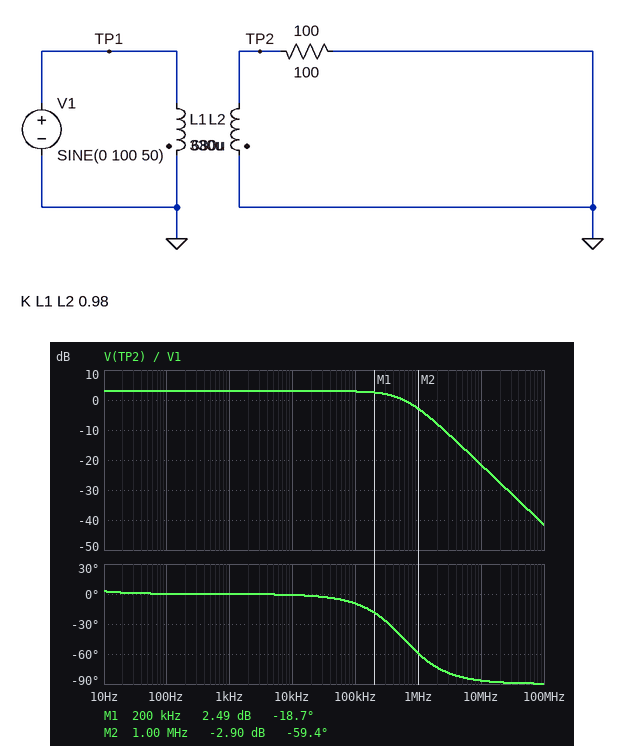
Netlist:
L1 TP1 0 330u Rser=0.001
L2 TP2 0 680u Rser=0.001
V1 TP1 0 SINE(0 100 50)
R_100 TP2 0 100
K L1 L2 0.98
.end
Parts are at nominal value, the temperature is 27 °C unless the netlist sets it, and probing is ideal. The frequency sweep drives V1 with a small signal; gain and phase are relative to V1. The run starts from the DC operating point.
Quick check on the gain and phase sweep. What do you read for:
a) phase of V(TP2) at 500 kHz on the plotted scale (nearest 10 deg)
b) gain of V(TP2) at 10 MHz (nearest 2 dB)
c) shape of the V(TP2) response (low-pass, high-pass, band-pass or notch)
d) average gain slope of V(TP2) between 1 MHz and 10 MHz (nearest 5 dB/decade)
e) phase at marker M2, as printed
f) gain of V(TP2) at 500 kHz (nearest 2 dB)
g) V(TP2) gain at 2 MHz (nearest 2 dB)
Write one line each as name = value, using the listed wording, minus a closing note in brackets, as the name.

phase of V(TP2) at 500 kHz on the plotted scale = -40 deg
gain of V(TP2) at 10 MHz = -22 dB
shape of the V(TP2) response = low-pass
average gain slope of V(TP2) between 1 MHz and 10 MHz = -20 dB/decade
phase at marker M2, as printed = -59.4 deg
gain of V(TP2) at 500 kHz = 0 dB
V(TP2) gain at 2 MHz = -8 dB
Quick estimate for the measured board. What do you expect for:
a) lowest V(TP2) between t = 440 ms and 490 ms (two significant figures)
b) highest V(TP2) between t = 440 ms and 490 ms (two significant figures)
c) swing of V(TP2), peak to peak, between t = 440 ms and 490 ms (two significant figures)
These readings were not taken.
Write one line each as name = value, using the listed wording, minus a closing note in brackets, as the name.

lowest V(TP2) between t = 440 ms and 490 ms = -140 V
highest V(TP2) between t = 440 ms and 490 ms = 140 V
swing of V(TP2), peak to peak, between t = 440 ms and 490 ms = 280 V
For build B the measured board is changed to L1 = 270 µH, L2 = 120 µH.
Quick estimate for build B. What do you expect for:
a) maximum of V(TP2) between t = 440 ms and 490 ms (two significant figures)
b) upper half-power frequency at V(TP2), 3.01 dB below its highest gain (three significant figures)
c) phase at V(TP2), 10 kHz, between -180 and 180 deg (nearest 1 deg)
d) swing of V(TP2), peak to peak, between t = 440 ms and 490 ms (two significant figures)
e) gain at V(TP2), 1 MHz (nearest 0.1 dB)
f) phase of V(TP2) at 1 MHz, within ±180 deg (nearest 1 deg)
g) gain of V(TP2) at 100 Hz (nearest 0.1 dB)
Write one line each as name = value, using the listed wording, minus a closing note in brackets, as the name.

maximum of V(TP2) between t = 440 ms and 490 ms = 65 V
upper half-power frequency at V(TP2), 3.01 dB below its highest gain = 3.35 MHz
phase at V(TP2), 10 kHz, between -180 and 180 deg = 0 deg
swing of V(TP2), peak to peak, between t = 440 ms and 490 ms = 130 V
gain at V(TP2), 1 MHz = -4.1 dB
phase of V(TP2) at 1 MHz, within ±180 deg = -17 deg
gain of V(TP2) at 100 Hz = -3.7 dB
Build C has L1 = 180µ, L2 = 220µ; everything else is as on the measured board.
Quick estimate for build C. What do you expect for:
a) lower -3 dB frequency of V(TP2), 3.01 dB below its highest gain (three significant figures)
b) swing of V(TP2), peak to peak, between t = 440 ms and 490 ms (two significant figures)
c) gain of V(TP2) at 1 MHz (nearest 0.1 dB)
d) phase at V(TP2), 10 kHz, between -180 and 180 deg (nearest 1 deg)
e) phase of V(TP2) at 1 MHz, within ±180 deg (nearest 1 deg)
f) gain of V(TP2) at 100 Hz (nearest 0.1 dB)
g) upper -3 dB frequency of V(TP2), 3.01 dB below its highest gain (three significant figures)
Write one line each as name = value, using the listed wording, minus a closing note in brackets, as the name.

lower -3 dB frequency of V(TP2), 3.01 dB below its highest gain = 884 mHz
swing of V(TP2), peak to peak, between t = 440 ms and 490 ms = 220 V
gain of V(TP2) at 1 MHz = -0.4 dB
phase at V(TP2), 10 kHz, between -180 and 180 deg = 0 deg
phase of V(TP2) at 1 MHz, within ±180 deg = -29 deg
gain of V(TP2) at 100 Hz = 0.7 dB
upper -3 dB frequency of V(TP2), 3.01 dB below its highest gain = 1.83 MHz
